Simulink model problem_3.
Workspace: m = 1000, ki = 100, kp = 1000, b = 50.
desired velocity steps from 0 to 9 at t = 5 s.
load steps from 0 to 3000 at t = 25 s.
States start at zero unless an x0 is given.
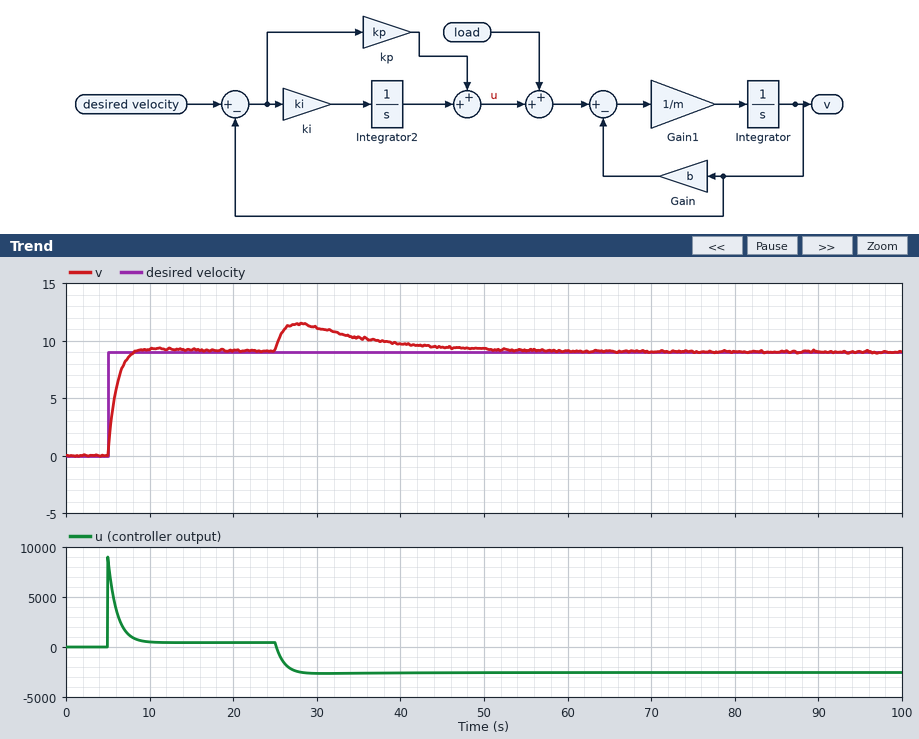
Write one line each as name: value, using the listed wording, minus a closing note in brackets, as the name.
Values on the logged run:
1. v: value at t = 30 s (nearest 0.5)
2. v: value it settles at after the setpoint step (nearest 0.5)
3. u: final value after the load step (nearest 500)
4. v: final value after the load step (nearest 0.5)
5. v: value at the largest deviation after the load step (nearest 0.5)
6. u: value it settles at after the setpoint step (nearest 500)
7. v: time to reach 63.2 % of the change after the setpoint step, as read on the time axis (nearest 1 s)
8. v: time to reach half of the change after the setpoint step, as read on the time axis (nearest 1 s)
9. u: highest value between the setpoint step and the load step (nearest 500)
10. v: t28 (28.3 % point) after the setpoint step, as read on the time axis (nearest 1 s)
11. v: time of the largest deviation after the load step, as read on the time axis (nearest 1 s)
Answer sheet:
v: value at t = 30 s: 11.0
v: value it settles at after the setpoint step: 9.0
u: final value after the load step: -2500
v: final value after the load step: 9.0
v: value at the largest deviation after the load step: 11.5
u: value it settles at after the setpoint step: 500
v: time to reach 63.2 % of the change after the setpoint step, as read on the time axis: 6 s
v: time to reach half of the change after the setpoint step, as read on the time axis: 6 s
u: highest value between the setpoint step and the load step: 9000
v: t28 (28.3 % point) after the setpoint step, as read on the time axis: 5 s
v: time of the largest deviation after the load step, as read on the time axis: 28 s
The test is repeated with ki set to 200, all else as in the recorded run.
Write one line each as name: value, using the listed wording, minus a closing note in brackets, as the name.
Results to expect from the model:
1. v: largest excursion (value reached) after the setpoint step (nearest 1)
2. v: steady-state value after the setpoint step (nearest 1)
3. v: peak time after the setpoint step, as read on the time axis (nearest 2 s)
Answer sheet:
v: largest excursion (value reached) after the setpoint step: 10
v: steady-state value after the setpoint step: 9
v: peak time after the setpoint step, as read on the time axis: 10 s
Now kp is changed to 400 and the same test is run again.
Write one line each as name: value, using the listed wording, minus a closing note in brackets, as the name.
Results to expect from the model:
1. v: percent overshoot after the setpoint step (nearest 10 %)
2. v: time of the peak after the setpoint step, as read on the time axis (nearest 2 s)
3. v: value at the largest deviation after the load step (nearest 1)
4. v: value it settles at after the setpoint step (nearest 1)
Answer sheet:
v: percent overshoot after the setpoint step: 20 %
v: time of the peak after the setpoint step, as read on the time axis: 12 s
v: value at the largest deviation after the load step: 13
v: value it settles at after the setpoint step: 9
